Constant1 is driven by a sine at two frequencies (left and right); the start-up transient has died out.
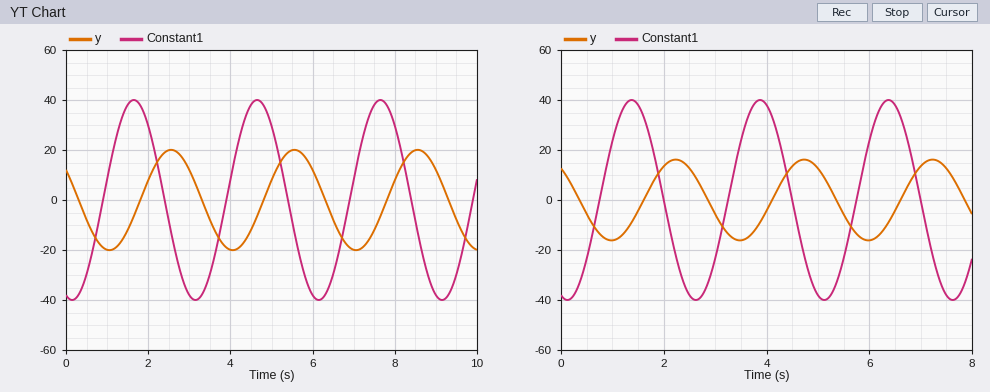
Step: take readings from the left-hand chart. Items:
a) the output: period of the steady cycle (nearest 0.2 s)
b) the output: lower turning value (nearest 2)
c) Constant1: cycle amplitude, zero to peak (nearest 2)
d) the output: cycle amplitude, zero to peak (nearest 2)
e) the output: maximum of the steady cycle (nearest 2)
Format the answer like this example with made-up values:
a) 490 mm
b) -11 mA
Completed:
a) 3.0 s
b) -20
c) 40
d) 20
e) 20
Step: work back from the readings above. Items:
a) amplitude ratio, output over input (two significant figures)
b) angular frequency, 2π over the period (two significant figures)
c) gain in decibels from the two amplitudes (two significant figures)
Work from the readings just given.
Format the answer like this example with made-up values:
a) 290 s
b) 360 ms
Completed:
a) 0.50
b) 2.1 rad/s
c) -6.0 dB
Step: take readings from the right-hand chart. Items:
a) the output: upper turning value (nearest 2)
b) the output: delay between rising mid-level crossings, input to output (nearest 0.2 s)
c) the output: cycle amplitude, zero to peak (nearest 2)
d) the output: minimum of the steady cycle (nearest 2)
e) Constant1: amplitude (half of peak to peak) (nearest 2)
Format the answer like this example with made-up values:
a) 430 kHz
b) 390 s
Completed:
a) 16
b) 0.8 s
c) 16
d) -16
e) 40
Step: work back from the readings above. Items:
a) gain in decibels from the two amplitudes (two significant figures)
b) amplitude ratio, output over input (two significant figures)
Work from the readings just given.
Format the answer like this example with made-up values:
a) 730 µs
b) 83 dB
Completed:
a) -8.0 dB
b) 0.40
